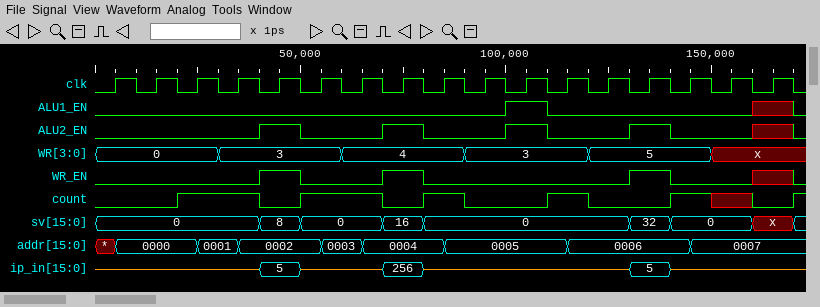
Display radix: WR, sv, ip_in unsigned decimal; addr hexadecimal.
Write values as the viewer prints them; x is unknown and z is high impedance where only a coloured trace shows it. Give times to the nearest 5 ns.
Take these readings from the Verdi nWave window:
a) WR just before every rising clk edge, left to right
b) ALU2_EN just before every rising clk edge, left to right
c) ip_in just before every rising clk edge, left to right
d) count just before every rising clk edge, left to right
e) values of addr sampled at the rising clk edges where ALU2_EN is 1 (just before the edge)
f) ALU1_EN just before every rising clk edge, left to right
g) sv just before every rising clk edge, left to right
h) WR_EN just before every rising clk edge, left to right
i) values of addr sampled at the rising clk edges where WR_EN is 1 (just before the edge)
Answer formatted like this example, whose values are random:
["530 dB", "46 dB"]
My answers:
["0, 0, 0, 3, 3, 3, 4, 4, 4, 3, 3, 3, 5, 5, 5, x, x", "0 0 0 0 1 0 0 1 0 0 1 0 0 1 0 0 x", "z, z, z, z, 5, z, z, 256, z, z, z, z, z, 5, z, z, z", "0 0 1 1 0 1 1 0 1 0 0 1 0 0 1 x 0", "0002, 0004, 0005, 0006", "0 0 0 0 0 0 0 0 0 0 1 0 0 0 0 0 x", "0, 0, 0, 0, 8, 0, 0, 16, 0, 0, 0, 0, 0, 32, 0, 0, x", "0 0 0 0 1 0 0 1 0 0 0 0 0 1 0 0 x", "0002, 0004, 0006"]
